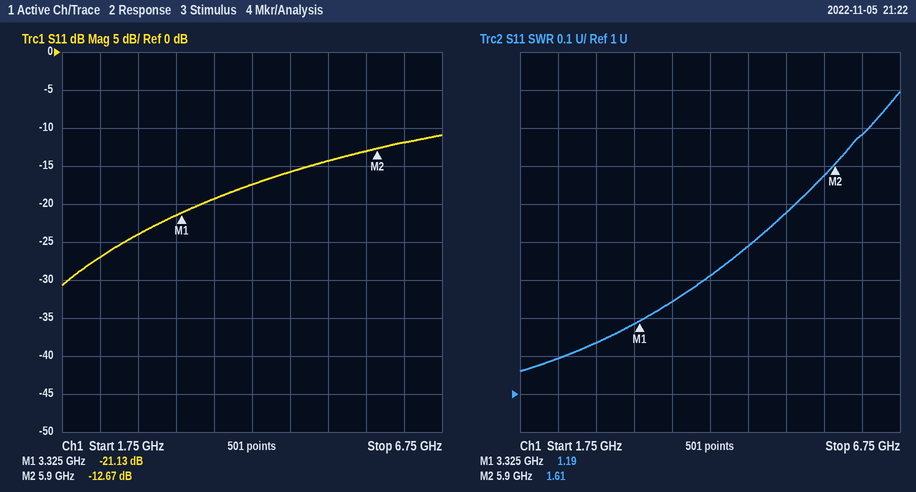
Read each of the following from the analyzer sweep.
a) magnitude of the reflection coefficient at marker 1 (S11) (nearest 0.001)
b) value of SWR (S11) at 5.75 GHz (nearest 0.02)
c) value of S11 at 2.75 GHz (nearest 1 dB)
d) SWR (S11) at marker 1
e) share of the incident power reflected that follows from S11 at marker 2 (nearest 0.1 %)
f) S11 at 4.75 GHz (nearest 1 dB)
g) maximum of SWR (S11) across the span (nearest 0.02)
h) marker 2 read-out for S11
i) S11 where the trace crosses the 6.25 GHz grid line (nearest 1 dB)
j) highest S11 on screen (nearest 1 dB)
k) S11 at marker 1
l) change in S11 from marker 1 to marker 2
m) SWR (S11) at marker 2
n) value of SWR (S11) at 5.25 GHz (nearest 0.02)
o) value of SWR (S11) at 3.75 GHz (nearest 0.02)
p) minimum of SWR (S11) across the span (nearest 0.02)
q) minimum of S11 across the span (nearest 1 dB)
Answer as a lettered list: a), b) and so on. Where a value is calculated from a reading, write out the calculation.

a) 10^(-21.13/20) ≈ 0.088
b) 1.58
c) -24 dB
d) 1.19
e) 10^(-12.67/10) ≈ 5.4 %
f) -16 dB
g) 1.80
h) -12.67 dB
i) -12 dB
j) -11 dB
k) -21.13 dB
l) -12.67 − (-21.13) = 8.46 dB
m) 1.61
n) 1.48
o) 1.24
p) 1.06
q) -31 dB
